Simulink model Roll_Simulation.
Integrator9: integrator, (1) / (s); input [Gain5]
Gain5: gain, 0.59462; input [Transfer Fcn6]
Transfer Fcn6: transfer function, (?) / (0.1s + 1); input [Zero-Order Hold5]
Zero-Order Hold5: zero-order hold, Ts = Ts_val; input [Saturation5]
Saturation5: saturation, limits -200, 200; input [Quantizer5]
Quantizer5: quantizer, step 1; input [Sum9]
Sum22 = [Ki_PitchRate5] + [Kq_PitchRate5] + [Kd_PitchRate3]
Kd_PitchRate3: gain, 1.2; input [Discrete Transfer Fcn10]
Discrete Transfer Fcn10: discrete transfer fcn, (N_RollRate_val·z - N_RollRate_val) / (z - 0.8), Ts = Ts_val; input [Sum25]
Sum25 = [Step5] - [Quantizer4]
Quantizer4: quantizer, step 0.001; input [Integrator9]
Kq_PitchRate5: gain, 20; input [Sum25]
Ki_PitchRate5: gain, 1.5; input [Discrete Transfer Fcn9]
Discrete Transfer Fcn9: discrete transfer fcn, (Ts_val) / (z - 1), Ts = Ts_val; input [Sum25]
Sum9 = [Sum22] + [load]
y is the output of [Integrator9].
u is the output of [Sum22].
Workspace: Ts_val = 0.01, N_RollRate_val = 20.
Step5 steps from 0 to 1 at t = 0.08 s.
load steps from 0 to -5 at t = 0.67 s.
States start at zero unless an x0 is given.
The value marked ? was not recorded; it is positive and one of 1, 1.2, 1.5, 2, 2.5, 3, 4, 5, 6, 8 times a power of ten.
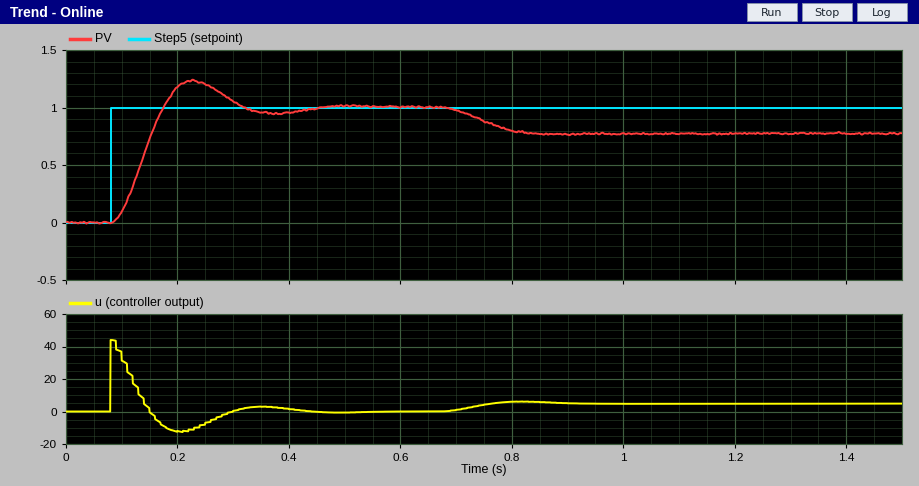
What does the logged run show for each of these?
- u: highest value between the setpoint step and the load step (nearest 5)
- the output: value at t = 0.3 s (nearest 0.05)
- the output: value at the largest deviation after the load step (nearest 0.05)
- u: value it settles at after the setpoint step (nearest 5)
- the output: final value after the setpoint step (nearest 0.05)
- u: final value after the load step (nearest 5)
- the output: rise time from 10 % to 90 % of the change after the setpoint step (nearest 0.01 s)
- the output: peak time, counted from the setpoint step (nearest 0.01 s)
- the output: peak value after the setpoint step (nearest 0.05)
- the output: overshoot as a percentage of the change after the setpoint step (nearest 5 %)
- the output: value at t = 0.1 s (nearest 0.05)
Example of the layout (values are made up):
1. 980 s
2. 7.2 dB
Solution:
1. 45
2. 1.05
3. 0.75
4. 0
5. 1.00
6. 5
7. 0.06 s
8. 0.15 s
9. 1.25
10. 25 %
11. 0.10
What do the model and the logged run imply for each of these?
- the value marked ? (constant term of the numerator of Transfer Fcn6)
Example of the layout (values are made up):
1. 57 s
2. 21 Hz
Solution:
1. 2
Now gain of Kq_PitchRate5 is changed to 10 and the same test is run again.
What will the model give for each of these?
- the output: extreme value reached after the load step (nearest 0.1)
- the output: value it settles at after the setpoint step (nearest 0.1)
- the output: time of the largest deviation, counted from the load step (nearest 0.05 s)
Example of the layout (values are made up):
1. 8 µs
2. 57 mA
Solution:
1. 0.6
2. 1.0
3. 0.85 s
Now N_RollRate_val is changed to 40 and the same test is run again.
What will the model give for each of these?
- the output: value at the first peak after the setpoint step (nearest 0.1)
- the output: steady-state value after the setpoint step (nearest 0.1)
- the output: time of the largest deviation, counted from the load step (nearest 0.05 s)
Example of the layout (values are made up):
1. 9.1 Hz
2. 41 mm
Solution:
1. 1.1
2. 1.0
3. 0.25 s
